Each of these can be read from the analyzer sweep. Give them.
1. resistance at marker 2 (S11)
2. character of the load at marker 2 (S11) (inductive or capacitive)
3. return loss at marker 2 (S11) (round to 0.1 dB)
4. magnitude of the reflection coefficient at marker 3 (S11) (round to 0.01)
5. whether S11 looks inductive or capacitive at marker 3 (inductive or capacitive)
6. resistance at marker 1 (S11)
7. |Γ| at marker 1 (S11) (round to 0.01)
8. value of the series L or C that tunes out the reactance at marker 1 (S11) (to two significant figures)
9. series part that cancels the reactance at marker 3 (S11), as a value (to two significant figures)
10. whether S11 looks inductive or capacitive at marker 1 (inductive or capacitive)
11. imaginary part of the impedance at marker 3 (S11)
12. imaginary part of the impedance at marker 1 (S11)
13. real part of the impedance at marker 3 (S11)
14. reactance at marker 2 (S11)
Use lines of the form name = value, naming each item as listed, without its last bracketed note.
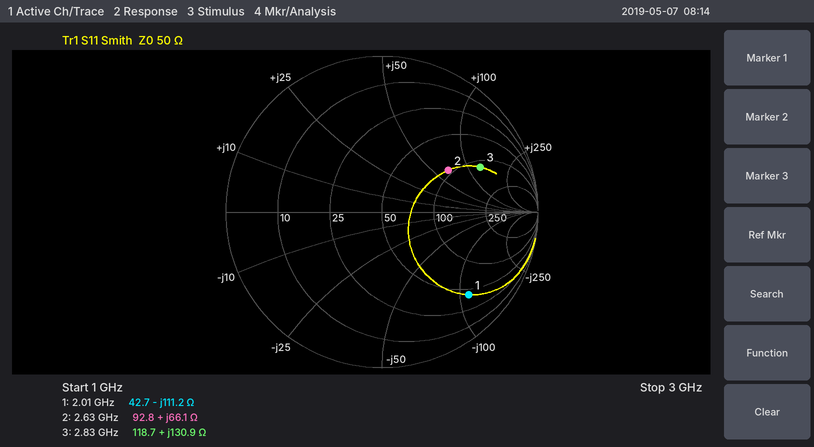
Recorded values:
resistance at marker 2 = 92.8 Ω
character of the load at marker 2 (S11) = inductive
return loss at marker 2 (S11) = 6.0 dB
magnitude of the reflection coefficient at marker 3 (S11) = 0.69
whether S11 looks inductive or capacitive at marker 3 = inductive
resistance at marker 1 = 42.7 Ω
|Γ| at marker 1 (S11) = 0.77
value of the series L or C that tunes out the reactance at marker 1 (S11) = 8.8 nH
series part that cancels the reactance at marker 3 (S11), as a value = 430 fF
whether S11 looks inductive or capacitive at marker 1 = capacitive
imaginary part of the impedance at marker 3 = +130.9 Ω
imaginary part of the impedance at marker 1 = -111.2 Ω
real part of the impedance at marker 3 = 118.7 Ω
reactance at marker 2 = +66.1 Ω
